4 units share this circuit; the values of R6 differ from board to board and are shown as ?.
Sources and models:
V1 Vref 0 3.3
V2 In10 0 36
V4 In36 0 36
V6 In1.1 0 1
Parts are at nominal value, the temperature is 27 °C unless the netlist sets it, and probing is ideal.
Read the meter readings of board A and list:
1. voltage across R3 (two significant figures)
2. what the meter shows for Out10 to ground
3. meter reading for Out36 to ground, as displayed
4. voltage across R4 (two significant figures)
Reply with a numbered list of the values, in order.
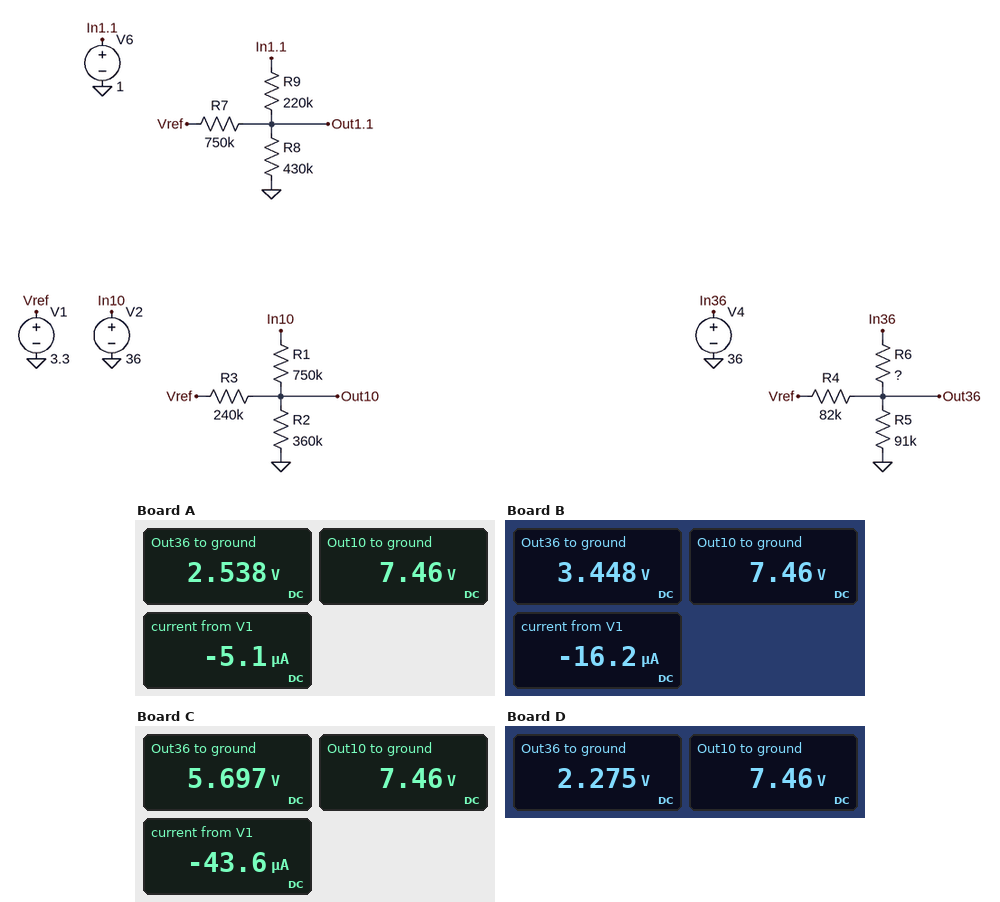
1. 4.2 V
2. 7.46 V
3. 2.538 V
4. 760 mV
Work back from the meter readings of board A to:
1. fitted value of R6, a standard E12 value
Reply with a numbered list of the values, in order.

1. 1.8 MΩ
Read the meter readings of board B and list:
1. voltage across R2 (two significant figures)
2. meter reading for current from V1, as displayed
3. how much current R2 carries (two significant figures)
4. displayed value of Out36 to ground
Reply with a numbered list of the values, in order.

1. 7.5 V
2. -16.2 µA
3. 21 µA
4. 3.448 V
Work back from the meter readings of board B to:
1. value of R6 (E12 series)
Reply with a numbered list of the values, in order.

1. 820 kΩ
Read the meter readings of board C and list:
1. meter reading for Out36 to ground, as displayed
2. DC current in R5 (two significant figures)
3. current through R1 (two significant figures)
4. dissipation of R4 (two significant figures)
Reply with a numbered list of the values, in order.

1. 5.697 V
2. 63 µA
3. 38 µA
4. 70 µW
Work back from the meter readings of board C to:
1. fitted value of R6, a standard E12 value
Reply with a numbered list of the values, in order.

1. 330 kΩ
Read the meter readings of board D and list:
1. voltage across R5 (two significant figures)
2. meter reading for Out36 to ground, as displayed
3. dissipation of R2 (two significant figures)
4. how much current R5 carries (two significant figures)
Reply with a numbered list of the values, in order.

1. 2.3 V
2. 2.275 V
3. 150 µW
4. 25 µA
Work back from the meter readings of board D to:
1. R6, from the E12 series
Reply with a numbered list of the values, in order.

1. 2.7 MΩ
